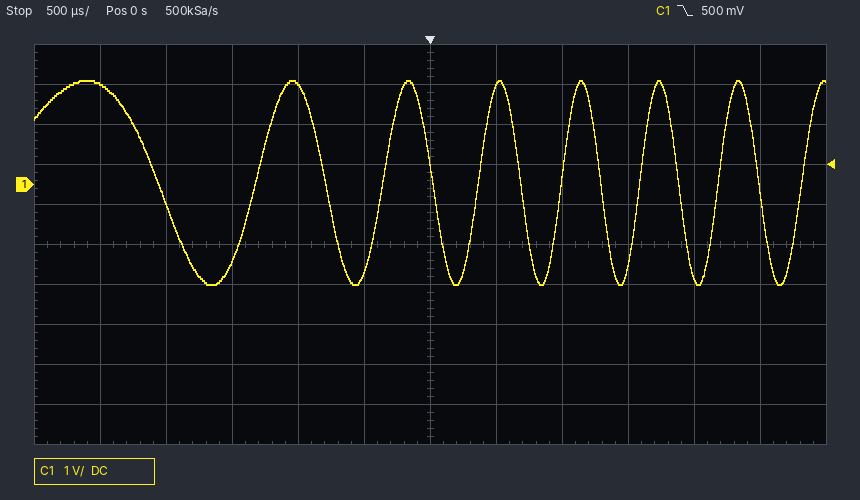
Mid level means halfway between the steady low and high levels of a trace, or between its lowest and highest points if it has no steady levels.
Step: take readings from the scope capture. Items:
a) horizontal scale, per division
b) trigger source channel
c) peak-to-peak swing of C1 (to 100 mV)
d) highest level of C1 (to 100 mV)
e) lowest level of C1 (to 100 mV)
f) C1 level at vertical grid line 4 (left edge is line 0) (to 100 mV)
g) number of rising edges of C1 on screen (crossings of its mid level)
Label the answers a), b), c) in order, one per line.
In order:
a) 500 µs
b) C1
c) 5.1 V
d) 2.6 V
e) -2.5 V
f) 2.5 V
g) 7
